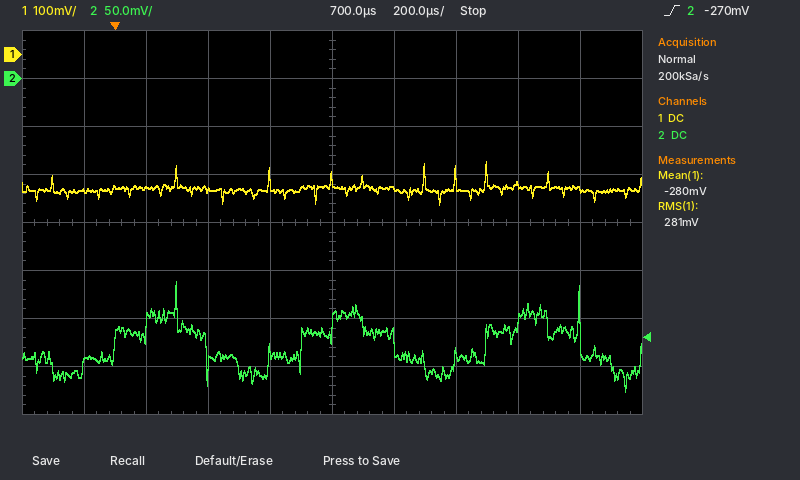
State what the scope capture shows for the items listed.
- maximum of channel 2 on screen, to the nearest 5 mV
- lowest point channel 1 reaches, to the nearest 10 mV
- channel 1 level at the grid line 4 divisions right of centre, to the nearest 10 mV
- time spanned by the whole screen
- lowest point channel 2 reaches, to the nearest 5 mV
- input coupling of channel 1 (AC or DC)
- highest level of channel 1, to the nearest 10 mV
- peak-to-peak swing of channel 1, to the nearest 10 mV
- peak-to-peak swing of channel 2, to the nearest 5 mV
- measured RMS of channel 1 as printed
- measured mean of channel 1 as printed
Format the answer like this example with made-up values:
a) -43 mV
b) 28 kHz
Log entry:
a) -210 mV
b) -310 mV
c) -280 mV
d) 2 ms
e) -325 mV
f) DC
g) -220 mV
h) 90 mV
i) 115 mV
j) 281 mV
k) -280 mV
